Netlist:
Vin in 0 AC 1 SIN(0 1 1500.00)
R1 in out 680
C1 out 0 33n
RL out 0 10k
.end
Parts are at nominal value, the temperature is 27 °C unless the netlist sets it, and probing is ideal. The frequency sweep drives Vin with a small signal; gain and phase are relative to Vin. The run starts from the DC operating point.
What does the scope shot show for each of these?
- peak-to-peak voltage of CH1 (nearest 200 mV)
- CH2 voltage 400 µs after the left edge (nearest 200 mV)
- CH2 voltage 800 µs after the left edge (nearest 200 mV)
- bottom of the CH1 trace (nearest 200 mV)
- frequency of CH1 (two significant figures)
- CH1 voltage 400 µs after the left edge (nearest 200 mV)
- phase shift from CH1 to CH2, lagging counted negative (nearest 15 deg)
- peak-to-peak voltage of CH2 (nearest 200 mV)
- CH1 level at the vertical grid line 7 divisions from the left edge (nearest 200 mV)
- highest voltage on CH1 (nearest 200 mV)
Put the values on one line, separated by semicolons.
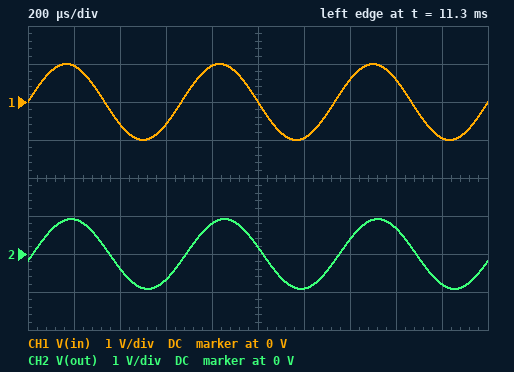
2.0 V; -400 mV; 800 mV; -1.0 V; 1.5 kHz; -600 mV; -15 deg; 1.8 V; 600 mV; 1.0 V
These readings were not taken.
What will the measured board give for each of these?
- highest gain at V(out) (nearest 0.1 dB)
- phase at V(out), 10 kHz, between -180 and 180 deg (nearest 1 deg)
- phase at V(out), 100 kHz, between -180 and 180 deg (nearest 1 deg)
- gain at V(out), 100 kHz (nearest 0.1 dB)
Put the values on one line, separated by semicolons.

-0.6 dB; -53 deg; -86 deg; -23.0 dB
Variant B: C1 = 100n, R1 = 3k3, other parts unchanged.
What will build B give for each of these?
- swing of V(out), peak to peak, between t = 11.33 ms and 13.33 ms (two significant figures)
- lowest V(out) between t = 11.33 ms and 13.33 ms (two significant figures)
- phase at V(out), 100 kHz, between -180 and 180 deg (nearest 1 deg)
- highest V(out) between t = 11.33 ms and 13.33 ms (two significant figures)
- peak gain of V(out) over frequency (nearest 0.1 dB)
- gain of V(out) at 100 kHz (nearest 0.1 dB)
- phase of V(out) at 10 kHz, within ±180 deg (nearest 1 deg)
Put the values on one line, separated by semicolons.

590 mV; -300 mV; -90 deg; 300 mV; -2.5 dB; -46.3 dB; -86 deg
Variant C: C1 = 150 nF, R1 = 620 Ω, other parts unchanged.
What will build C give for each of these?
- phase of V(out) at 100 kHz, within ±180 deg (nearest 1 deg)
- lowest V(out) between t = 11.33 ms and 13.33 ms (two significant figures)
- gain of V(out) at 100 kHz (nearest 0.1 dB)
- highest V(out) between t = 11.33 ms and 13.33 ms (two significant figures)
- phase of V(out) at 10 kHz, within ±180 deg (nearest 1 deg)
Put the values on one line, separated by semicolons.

-89 deg; -730 mV; -35.3 dB; 730 mV; -80 deg
